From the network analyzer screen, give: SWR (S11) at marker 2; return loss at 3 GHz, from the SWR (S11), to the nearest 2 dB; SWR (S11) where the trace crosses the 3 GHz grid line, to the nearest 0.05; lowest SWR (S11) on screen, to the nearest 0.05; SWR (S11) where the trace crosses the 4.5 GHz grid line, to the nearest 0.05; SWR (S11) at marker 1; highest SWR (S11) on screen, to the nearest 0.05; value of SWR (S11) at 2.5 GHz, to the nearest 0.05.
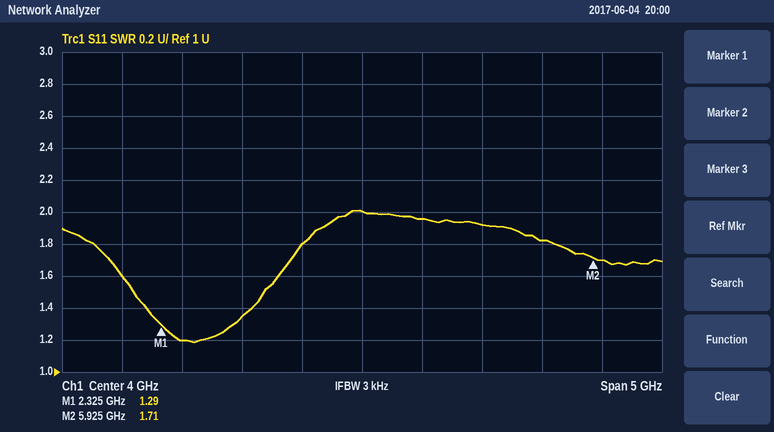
1.71
16 dB
1.35
1.20
1.95
1.29
2.00
1.20
